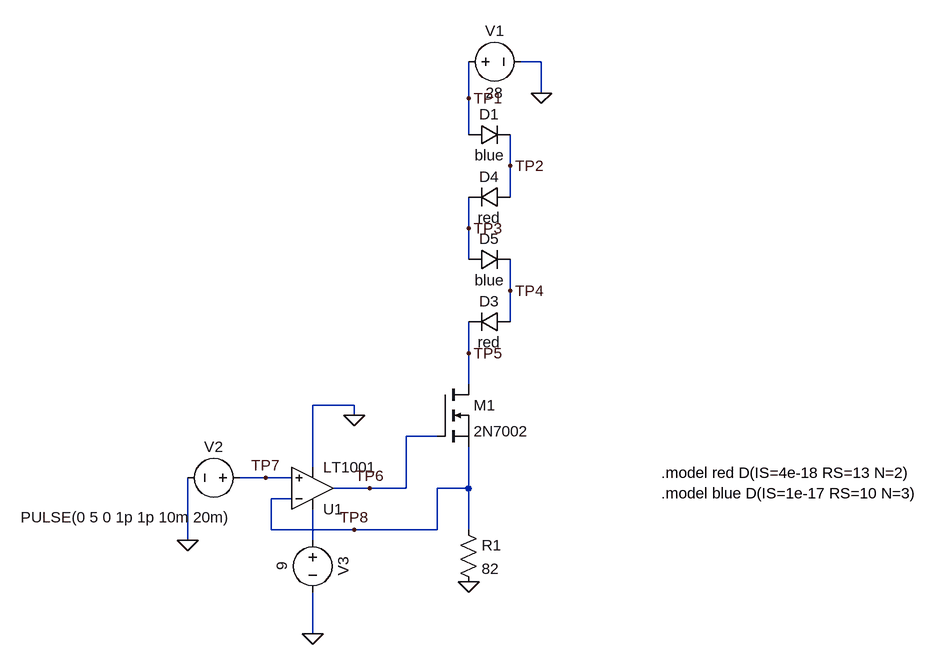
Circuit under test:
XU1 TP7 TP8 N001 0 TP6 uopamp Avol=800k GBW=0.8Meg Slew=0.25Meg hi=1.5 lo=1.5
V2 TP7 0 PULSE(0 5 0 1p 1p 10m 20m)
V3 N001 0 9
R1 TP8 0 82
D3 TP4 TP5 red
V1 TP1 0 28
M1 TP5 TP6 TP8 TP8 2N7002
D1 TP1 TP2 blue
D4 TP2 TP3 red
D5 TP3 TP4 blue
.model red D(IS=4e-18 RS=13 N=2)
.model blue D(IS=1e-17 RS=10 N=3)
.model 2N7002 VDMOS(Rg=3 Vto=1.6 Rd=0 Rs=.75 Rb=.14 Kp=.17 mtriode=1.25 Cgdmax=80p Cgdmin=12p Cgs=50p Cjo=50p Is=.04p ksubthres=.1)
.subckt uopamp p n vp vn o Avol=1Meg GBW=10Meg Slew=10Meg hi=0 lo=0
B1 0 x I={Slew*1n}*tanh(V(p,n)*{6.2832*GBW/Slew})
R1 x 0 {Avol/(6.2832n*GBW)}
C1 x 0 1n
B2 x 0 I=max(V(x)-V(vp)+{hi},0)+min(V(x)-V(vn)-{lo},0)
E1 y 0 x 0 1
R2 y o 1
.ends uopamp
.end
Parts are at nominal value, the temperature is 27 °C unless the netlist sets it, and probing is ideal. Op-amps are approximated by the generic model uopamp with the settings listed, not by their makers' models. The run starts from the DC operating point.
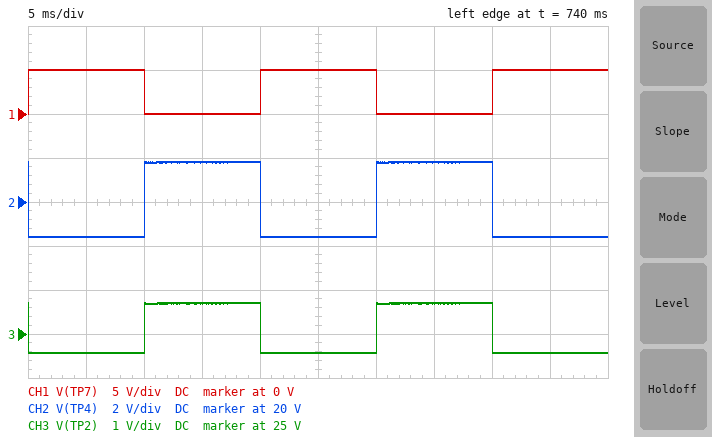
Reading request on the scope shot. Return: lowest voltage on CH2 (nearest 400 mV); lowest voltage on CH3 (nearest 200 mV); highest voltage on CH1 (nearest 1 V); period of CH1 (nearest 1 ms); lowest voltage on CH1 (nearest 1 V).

18.4 V
24.6 V
5 V
20 ms
0 V
